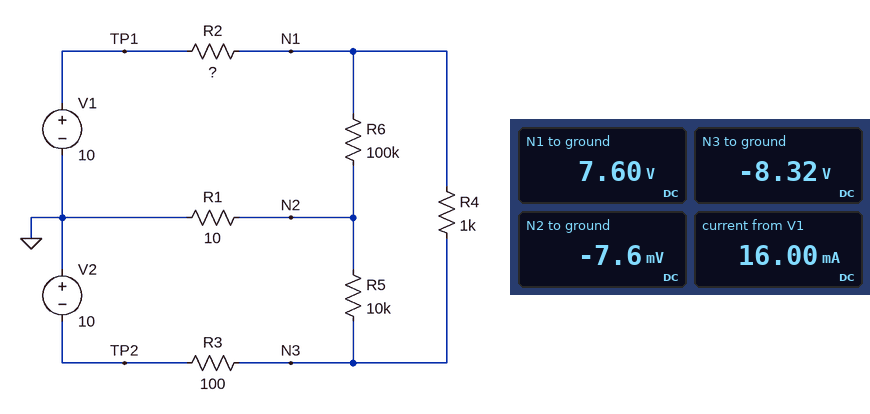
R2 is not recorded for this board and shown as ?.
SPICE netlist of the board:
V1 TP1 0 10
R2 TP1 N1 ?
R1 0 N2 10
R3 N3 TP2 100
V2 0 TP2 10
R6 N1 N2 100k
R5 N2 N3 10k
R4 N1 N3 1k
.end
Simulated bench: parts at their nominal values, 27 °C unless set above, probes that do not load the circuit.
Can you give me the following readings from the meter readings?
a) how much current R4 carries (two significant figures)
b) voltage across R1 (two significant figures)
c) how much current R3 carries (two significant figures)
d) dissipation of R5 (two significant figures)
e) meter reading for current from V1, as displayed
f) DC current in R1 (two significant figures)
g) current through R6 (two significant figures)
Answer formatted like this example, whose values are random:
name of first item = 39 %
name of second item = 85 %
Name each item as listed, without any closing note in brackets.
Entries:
how much current R4 carries = 16 mA
voltage across R1 = 7.6 mV
how much current R3 carries = 17 mA
dissipation of R5 = 6.9 mW
meter reading for current from V1, as displayed = 16.00 mA
DC current in R1 = 760 µA
current through R6 = 76 µA
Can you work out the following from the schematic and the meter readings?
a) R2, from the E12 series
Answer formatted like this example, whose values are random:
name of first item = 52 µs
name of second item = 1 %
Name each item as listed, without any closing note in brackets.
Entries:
R2, from the E12 series = 150 Ω
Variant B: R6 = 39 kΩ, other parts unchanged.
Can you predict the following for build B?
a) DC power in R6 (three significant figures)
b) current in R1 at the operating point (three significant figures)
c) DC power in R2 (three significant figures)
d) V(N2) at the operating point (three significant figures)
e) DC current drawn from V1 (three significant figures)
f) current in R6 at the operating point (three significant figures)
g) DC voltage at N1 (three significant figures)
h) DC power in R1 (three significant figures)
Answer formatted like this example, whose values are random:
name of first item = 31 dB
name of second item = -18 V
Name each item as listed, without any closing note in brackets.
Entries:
DC power in R6 = 1.48 mW
current in R1 at the operating point = 637 µA
DC power in R2 = 38.9 mW
V(N2) at the operating point = -6.37 mV
DC current drawn from V1 = 16.1 mA
current in R6 at the operating point = 195 µA
DC voltage at N1 = 7.58 V
DC power in R1 = 4.06 µW
